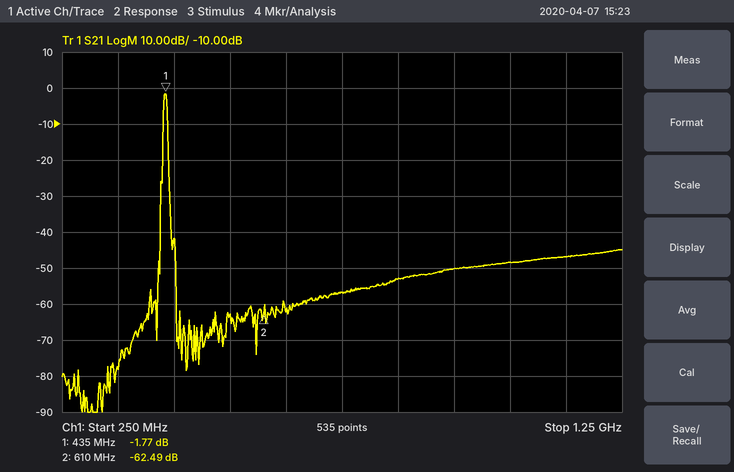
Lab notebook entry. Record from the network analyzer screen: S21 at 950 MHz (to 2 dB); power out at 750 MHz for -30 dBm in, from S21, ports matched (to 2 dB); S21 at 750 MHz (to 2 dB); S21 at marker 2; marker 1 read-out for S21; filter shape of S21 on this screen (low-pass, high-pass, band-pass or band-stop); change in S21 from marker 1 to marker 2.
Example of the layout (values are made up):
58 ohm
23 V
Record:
-50 dB
-86 dBm
-56 dB
-62.49 dB
-1.77 dB
band-pass
-60.72 dB
